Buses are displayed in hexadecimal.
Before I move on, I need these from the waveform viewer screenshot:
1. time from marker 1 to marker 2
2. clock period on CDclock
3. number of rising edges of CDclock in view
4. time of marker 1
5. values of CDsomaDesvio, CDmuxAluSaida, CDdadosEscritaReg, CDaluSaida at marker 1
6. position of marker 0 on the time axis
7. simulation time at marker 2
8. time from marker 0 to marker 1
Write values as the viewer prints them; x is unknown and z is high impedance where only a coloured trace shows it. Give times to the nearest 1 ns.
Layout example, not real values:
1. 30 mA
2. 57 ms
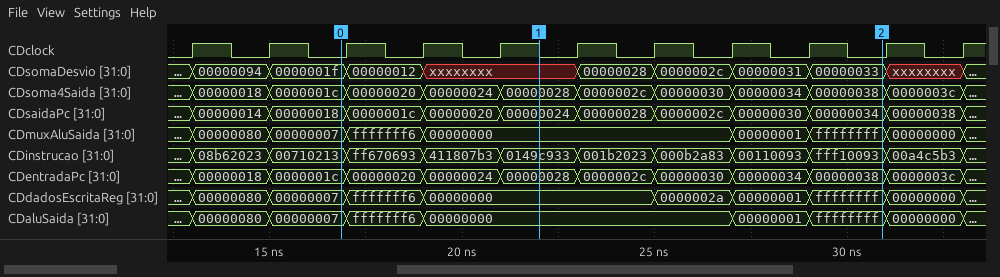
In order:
1. 9 ns
2. 2 ns
3. 11
4. 22 ns
5. CDsomaDesvio=xxxxxxxx, CDmuxAluSaida=00000000, CDdadosEscritaReg=00000000, CDaluSaida=00000000
6. 17 ns
7. 31 ns
8. 5 ns
